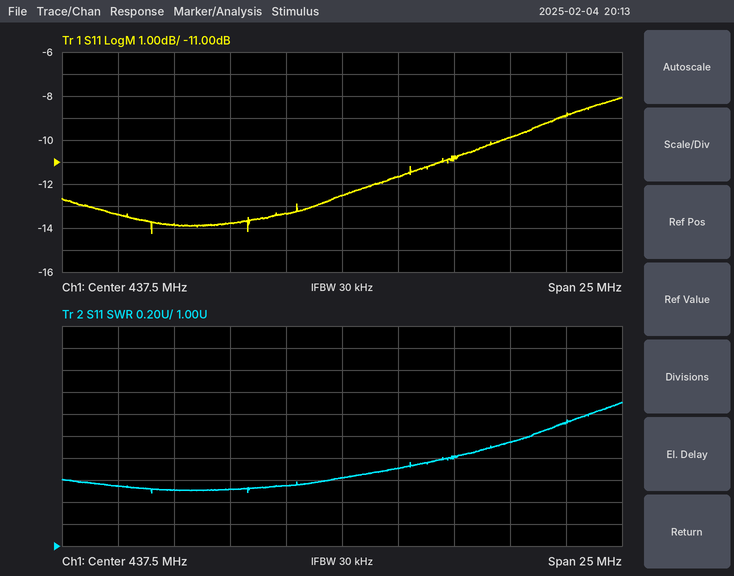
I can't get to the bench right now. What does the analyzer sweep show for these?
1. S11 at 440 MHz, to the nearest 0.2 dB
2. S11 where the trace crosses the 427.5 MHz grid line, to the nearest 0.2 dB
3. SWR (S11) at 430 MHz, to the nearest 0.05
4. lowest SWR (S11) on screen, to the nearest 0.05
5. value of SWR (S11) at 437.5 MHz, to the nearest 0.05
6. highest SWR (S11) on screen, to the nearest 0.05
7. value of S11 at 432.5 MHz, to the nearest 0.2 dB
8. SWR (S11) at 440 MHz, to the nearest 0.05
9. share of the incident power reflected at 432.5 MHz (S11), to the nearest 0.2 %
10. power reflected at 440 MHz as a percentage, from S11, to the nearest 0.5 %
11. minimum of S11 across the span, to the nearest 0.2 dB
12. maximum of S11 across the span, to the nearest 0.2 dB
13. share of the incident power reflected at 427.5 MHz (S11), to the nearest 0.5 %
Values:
-11.6 dB
-13.4 dB
1.50
1.50
1.60
2.30
-13.8 dB
1.70
4.2 %
7.0 %
-14.2 dB
-8.0 dB
4.5 %
